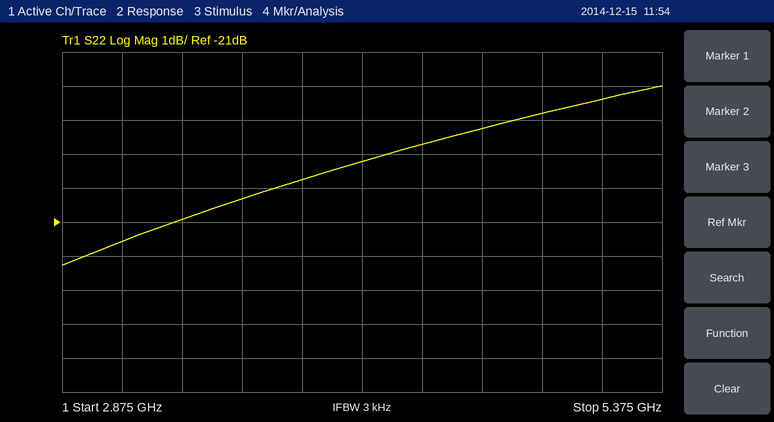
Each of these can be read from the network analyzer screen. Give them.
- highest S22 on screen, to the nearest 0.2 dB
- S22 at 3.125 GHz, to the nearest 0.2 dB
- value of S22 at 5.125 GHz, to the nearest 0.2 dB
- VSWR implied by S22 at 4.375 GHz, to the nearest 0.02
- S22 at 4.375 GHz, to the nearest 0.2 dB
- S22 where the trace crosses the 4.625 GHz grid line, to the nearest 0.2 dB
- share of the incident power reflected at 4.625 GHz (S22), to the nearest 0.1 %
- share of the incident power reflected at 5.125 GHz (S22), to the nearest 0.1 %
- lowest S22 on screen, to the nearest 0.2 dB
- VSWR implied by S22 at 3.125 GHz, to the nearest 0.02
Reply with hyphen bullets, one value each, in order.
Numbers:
- -17.0 dB
- -21.6 dB
- -17.4 dB
- 1.26
- -18.8 dB
- -18.2 dB
- 1.5 %
- 1.8 %
- -22.2 dB
- 1.18
